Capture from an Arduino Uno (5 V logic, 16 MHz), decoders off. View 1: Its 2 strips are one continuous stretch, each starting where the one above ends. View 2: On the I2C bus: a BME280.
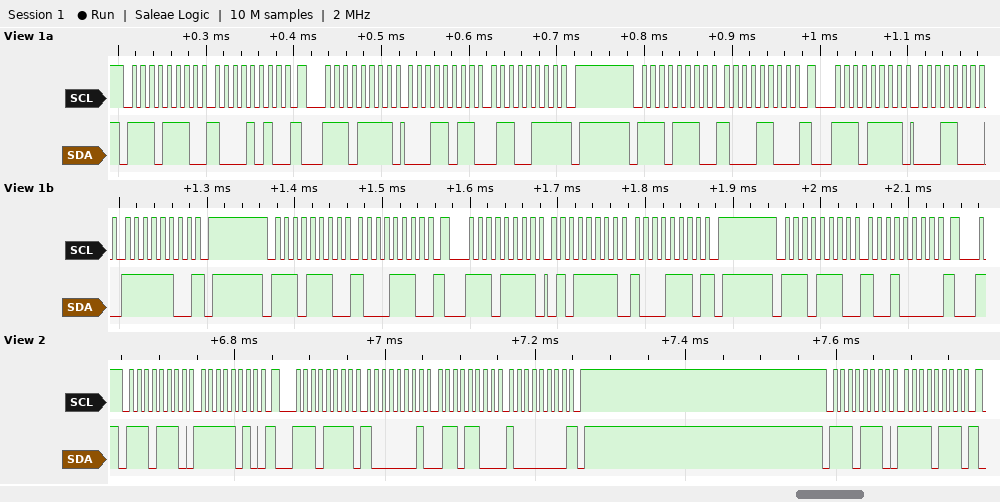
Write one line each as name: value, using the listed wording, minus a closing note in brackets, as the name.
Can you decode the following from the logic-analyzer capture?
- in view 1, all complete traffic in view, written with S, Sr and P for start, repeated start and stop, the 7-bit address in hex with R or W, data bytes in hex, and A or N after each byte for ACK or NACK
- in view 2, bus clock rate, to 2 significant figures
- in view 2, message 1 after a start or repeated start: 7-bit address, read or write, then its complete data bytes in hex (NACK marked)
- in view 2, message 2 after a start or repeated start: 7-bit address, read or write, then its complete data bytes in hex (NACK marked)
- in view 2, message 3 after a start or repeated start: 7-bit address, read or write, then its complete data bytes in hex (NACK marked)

in view 1, all complete traffic in view, written with S, Sr and P for start, repeated start and stop, the 7-bit address in hex with R or W, data bytes in hex, and A or N after each byte for ACK or NACK: S 77W A 8A A Sr 77R A 1B A 67 N P S 77W A 8C A Sr 77R A 18 A FC N P S 77W A 8E A Sr 77R A 5F A 8E N P S 77W A 90 A
in view 2, bus clock rate, to 2 significant figures: 100 kHz
in view 2, message 1 after a start or repeated start: 7-bit address, read or write, then its complete data bytes in hex: 0x77 write: FA
in view 2, message 2 after a start or repeated start: 7-bit address, read or write, then its complete data bytes in hex: 0x77 read: 81 6C 80 NACK
in view 2, message 3 after a start or repeated start: 7-bit address, read or write, then its complete data bytes in hex: 0x77 write: F7
